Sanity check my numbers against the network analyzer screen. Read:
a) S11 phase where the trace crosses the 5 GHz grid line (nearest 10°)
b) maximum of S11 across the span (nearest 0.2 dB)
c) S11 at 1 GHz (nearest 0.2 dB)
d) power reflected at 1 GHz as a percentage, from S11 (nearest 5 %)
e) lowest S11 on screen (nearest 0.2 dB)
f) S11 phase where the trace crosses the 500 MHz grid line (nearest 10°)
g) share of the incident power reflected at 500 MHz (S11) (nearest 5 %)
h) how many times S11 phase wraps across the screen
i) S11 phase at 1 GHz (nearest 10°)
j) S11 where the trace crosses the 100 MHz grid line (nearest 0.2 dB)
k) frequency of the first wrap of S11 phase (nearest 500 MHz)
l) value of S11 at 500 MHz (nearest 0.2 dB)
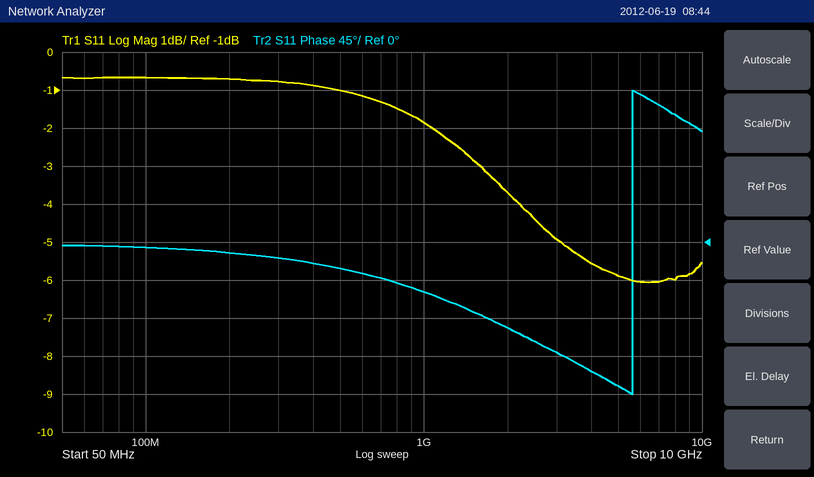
-170°
-0.6 dB
-1.8 dB
65 %
-6.0 dB
-30°
80 %
1
-60°
-0.6 dB
5.5 GHz
-1.0 dB
